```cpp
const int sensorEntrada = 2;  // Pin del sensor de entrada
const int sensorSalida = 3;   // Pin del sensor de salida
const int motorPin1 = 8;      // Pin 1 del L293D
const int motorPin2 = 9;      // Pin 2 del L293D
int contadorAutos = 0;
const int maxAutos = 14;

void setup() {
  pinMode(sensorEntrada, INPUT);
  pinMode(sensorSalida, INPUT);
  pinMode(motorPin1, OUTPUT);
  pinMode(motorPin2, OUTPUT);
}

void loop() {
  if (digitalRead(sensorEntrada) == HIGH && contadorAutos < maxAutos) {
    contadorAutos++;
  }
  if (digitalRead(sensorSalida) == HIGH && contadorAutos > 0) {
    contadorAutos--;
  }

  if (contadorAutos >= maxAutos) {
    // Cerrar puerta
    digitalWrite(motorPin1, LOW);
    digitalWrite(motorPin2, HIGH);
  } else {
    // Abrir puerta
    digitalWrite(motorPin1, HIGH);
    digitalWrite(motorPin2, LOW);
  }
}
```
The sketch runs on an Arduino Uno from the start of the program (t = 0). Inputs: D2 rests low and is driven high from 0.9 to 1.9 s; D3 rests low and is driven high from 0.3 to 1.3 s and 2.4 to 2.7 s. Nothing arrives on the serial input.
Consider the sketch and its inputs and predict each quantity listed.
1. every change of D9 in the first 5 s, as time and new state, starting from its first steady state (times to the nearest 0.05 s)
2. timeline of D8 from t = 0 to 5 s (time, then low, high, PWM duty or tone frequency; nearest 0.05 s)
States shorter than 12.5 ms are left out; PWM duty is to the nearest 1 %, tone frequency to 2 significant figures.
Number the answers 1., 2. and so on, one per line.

1. 0 s low; 1.3 s high; 2.4 s low
2. 0 s high; 1.3 s low; 2.4 s high
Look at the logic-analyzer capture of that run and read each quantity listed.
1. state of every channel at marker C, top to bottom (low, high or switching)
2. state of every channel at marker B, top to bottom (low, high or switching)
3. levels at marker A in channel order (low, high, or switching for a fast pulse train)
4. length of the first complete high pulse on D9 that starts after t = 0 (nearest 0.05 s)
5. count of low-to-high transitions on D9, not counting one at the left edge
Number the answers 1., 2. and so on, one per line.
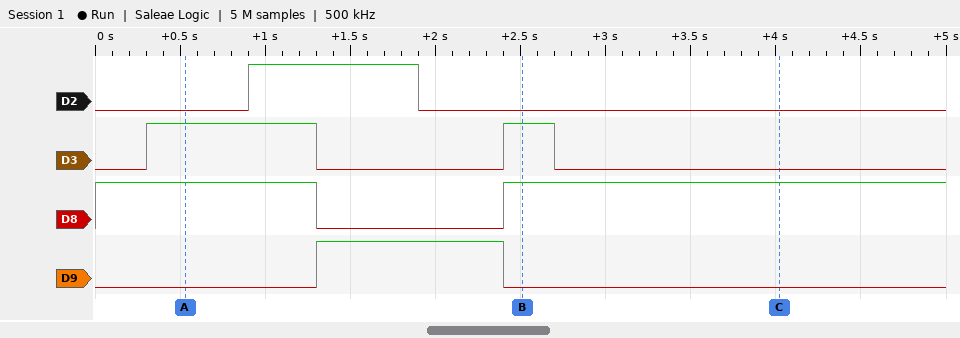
1. D2 low, D3 low, D8 high, D9 low
2. D2 low, D3 high, D8 high, D9 low
3. D2 low, D3 high, D8 high, D9 low
4. 1.10 s
5. 1
